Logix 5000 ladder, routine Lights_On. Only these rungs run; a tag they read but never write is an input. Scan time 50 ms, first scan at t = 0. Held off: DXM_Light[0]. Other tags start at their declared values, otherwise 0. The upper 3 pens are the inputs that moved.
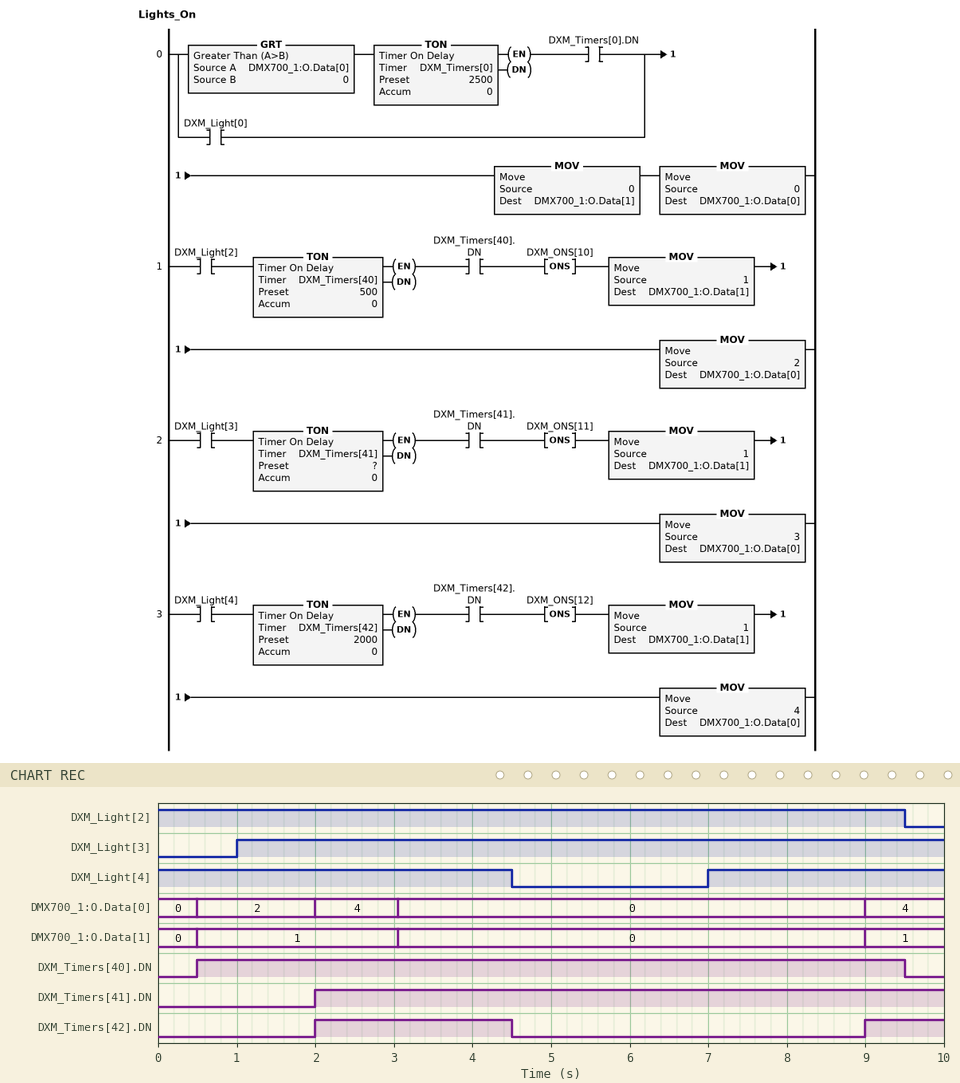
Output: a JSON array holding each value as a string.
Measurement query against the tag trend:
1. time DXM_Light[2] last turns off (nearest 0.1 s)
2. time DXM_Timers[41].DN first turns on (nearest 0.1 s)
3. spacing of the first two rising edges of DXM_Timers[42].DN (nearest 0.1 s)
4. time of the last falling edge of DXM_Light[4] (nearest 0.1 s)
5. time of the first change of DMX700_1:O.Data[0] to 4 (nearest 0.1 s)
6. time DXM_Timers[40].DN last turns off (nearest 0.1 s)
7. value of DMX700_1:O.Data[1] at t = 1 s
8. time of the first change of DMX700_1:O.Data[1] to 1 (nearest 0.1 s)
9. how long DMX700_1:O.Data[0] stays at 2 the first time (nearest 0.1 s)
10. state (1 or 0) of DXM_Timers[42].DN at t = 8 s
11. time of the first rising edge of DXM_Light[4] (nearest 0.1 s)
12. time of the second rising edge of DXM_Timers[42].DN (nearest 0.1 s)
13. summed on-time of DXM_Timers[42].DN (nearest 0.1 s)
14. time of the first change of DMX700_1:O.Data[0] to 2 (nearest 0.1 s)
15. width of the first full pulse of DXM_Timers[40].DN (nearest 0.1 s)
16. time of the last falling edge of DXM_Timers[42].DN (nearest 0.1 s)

["9.5 s", "2.0 s", "7.0 s", "4.5 s", "2.0 s", "9.5 s", "1", "0.5 s", "1.5 s", "0", "7.0 s", "9.0 s", "3.5 s", "0.5 s", "9.0 s", "4.5 s"]
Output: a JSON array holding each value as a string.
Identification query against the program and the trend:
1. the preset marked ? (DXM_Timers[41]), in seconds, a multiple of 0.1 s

["1.0 s"]
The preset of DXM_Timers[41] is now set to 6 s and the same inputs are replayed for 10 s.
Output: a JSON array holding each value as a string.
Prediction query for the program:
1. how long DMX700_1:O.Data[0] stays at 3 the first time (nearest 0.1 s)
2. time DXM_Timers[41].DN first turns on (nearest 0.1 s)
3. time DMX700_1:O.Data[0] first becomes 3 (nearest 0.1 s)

["2.0 s", "7.0 s", "7.0 s"]
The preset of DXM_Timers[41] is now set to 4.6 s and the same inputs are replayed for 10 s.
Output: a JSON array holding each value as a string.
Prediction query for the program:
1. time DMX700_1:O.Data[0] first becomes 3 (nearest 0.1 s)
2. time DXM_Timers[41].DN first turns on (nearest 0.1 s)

["5.6 s", "5.6 s"]
